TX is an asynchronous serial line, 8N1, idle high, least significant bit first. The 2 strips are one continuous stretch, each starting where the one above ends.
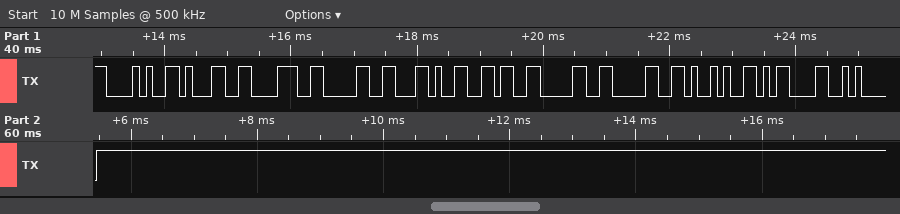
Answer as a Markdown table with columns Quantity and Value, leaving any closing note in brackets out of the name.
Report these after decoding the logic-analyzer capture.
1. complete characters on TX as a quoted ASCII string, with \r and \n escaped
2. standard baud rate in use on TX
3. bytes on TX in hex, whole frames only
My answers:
| Quantity | Value |
|---|---|
| complete characters on TX as a quoted ASCII string, with \r and \n escaped | "(180,600)\r\n" |
| standard baud rate in use on TX | 9600 baud |
| bytes on TX in hex, whole frames only | 0x28 0x31 0x38 0x30 0x2C 0x36 0x30 0x30 0x29 0x0D 0x0A |
